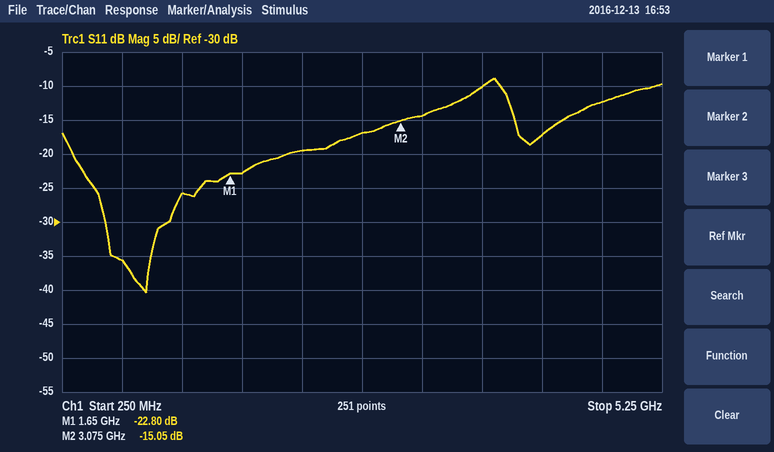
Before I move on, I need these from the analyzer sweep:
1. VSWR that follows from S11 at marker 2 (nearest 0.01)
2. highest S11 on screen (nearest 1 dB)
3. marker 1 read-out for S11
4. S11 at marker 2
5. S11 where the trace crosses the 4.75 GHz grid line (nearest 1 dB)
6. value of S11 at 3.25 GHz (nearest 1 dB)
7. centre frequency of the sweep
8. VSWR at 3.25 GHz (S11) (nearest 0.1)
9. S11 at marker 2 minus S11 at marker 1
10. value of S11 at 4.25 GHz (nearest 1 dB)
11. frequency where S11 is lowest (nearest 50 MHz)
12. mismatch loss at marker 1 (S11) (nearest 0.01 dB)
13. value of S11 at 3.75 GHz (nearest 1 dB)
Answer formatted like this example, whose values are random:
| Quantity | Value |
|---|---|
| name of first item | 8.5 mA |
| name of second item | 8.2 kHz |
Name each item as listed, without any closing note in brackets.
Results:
| Quantity | Value |
|---|---|
| VSWR that follows from S11 at marker 2 | 1.43 |
| highest S11 on screen | -9 dB |
| marker 1 read-out for S11 | -22.80 dB |
| S11 at marker 2 | -15.05 dB |
| S11 where the trace crosses the 4.75 GHz grid line | -12 dB |
| value of S11 at 3.25 GHz | -14 dB |
| centre frequency of the sweep | 2.75 GHz |
| VSWR at 3.25 GHz (S11) | 1.5 |
| S11 at marker 2 minus S11 at marker 1 | 7.75 dB |
| value of S11 at 4.25 GHz | -17 dB |
| frequency where S11 is lowest | 950 MHz |
| mismatch loss at marker 1 (S11) | 0.02 dB |
| value of S11 at 3.75 GHz | -10 dB |
